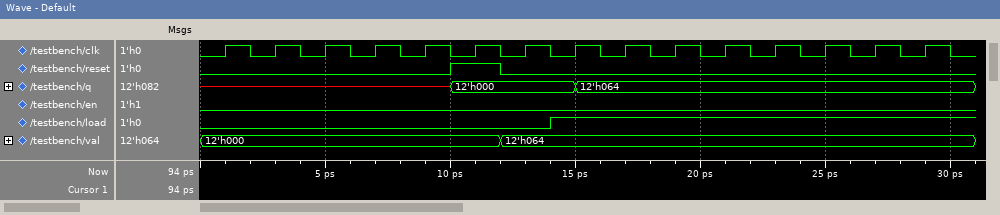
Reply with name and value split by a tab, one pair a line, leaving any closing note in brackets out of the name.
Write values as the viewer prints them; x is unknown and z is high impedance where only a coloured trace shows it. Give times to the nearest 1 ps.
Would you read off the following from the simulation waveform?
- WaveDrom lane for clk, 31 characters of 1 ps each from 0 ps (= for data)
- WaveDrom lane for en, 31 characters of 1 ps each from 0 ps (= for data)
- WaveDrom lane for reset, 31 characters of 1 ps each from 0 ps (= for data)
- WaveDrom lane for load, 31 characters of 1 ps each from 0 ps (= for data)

WaveDrom lane for clk, 31 characters of 1 ps each from 0 ps	{name: 'clk', wave: '0101010101010101010101010101010'}
WaveDrom lane for en, 31 characters of 1 ps each from 0 ps	{name: 'en', wave: '0..............................'}
WaveDrom lane for reset, 31 characters of 1 ps each from 0 ps	{name: 'reset', wave: '0.........1.0..................'}
WaveDrom lane for load, 31 characters of 1 ps each from 0 ps	{name: 'load', wave: '0.............1................'}
